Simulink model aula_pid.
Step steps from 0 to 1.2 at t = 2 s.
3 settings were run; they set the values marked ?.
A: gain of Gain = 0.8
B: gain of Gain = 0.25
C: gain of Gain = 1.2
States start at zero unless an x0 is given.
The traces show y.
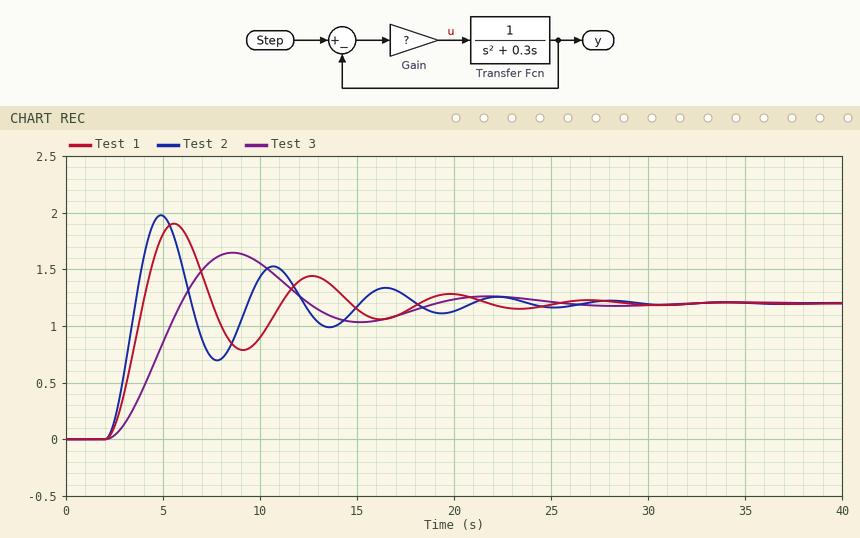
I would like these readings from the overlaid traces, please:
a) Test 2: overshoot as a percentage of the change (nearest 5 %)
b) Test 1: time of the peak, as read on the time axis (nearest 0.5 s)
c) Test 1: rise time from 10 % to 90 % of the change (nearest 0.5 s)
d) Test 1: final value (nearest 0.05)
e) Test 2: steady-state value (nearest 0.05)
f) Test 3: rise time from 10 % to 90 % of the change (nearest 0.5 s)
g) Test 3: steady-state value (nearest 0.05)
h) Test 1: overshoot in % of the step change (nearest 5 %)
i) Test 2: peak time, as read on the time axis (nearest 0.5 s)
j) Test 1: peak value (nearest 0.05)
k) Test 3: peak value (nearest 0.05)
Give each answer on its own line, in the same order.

65 %
5.5 s
1.5 s
1.20
1.20
2.5 s
1.20
60 %
5.0 s
1.90
1.65
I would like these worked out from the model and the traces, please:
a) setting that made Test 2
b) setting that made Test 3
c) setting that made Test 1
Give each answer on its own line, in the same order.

C
B
A
